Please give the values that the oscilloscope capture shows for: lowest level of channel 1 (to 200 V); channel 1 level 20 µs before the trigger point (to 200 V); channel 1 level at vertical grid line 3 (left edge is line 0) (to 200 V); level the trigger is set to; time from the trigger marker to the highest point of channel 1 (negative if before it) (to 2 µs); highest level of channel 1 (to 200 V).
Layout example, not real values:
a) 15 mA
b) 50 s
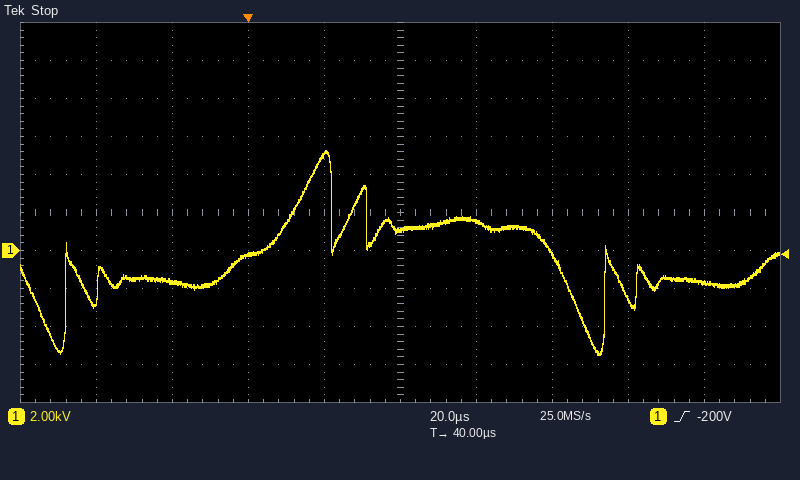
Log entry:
a) -5.4 kV
b) -1.6 kV
c) -200 V
d) -200 V
e) +20 µs
f) 5.2 kV
